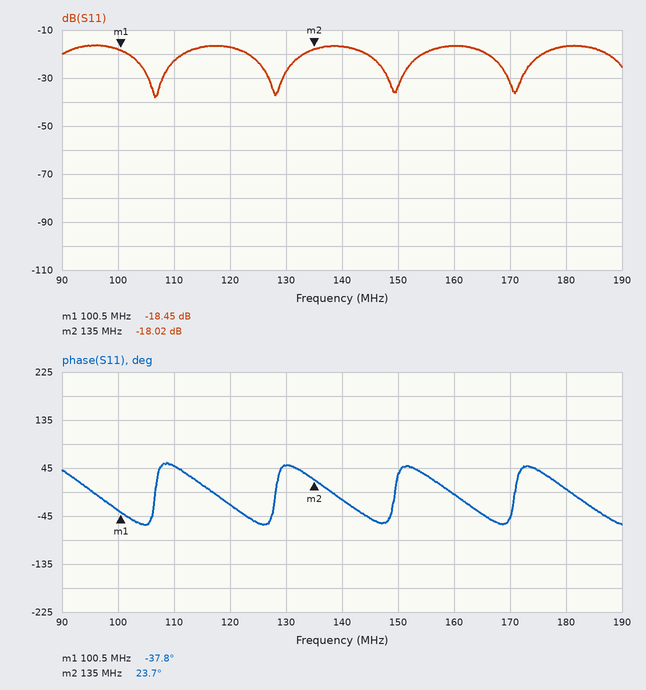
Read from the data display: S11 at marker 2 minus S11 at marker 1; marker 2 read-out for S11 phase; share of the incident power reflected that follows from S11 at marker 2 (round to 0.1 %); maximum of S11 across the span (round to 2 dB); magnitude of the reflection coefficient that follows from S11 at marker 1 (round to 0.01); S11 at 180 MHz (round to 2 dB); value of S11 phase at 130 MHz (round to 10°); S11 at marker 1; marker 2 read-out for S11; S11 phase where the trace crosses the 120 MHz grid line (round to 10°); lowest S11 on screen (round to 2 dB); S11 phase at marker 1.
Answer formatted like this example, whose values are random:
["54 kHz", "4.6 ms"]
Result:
["0.43 dB", "23.7°", "1.6 %", "-16 dB", "0.12", "-16 dB", "50°", "-18.45 dB", "-18.02 dB", "-20°", "-38 dB", "-37.8°"]
